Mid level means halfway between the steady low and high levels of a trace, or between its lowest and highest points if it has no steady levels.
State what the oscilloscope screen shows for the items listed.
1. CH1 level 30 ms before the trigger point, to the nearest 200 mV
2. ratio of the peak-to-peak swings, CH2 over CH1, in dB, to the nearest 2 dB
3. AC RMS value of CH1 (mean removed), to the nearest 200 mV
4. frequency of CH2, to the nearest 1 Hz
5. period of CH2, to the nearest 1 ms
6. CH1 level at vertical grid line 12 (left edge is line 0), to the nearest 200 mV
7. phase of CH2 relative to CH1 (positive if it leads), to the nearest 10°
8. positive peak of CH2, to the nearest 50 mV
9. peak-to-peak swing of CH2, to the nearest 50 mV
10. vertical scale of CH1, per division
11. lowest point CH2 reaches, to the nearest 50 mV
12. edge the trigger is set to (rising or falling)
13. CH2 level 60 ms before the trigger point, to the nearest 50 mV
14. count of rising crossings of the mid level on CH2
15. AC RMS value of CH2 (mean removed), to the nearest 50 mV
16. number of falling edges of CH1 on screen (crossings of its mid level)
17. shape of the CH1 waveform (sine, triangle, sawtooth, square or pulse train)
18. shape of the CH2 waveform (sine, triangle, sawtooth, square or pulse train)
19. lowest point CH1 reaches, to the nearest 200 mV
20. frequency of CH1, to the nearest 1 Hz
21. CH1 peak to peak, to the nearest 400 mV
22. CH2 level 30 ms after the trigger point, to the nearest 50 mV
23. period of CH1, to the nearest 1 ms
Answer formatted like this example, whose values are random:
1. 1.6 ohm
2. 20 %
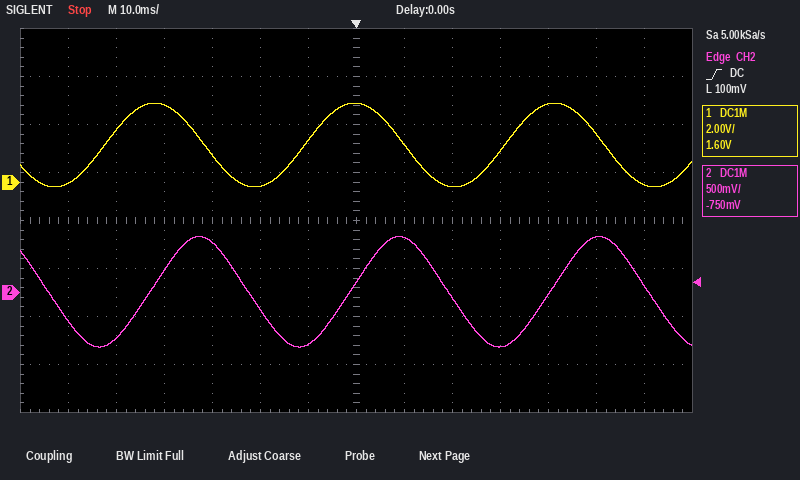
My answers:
1. 1.2 V
2. -10 dB
3. 1.2 V
4. 24 Hz
5. 42 ms
6. 2.0 V
7. -80°
8. 600 mV
9. 1.15 V
10. 2 V
11. -550 mV
12. rising
13. -300 mV
14. 3
15. 400 mV
16. 3
17. sine
18. sine
19. -200 mV
20. 24 Hz
21. 3.6 V
22. -550 mV
23. 42 ms
